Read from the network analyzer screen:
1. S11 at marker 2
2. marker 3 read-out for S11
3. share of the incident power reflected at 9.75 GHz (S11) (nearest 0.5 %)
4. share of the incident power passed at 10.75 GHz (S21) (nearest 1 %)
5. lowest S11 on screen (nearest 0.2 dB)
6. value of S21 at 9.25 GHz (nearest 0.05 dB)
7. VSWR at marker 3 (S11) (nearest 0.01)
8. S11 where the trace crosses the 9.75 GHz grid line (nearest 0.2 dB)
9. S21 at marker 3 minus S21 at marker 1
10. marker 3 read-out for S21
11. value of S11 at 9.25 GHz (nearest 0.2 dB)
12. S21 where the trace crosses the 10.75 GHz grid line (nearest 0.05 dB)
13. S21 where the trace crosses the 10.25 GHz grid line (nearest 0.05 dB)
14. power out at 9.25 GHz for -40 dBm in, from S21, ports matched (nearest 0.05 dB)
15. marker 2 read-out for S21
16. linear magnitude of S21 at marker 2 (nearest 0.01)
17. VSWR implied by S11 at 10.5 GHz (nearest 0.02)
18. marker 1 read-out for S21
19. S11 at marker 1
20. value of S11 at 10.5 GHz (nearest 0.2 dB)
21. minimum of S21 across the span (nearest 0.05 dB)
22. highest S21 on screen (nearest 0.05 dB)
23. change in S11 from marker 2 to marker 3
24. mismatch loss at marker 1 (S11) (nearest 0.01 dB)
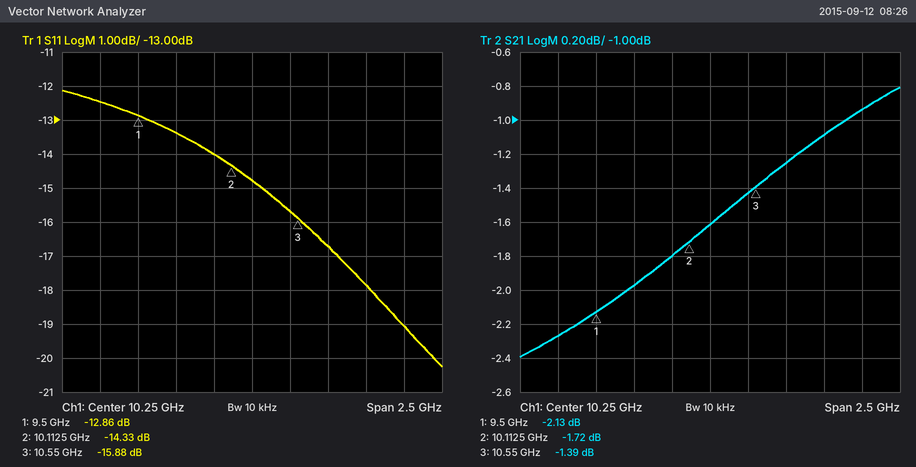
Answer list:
-14.33 dB
-15.88 dB
4.5 %
75 %
-20.2 dB
-2.25 dB
1.38
-13.4 dB
0.74 dB
-1.39 dB
-12.4 dB
-1.25 dB
-1.60 dB
-42.25 dBm
-1.72 dB
0.82
1.40
-2.13 dB
-12.86 dB
-15.6 dB
-2.40 dB
-0.80 dB
-1.55 dB
0.23 dB
